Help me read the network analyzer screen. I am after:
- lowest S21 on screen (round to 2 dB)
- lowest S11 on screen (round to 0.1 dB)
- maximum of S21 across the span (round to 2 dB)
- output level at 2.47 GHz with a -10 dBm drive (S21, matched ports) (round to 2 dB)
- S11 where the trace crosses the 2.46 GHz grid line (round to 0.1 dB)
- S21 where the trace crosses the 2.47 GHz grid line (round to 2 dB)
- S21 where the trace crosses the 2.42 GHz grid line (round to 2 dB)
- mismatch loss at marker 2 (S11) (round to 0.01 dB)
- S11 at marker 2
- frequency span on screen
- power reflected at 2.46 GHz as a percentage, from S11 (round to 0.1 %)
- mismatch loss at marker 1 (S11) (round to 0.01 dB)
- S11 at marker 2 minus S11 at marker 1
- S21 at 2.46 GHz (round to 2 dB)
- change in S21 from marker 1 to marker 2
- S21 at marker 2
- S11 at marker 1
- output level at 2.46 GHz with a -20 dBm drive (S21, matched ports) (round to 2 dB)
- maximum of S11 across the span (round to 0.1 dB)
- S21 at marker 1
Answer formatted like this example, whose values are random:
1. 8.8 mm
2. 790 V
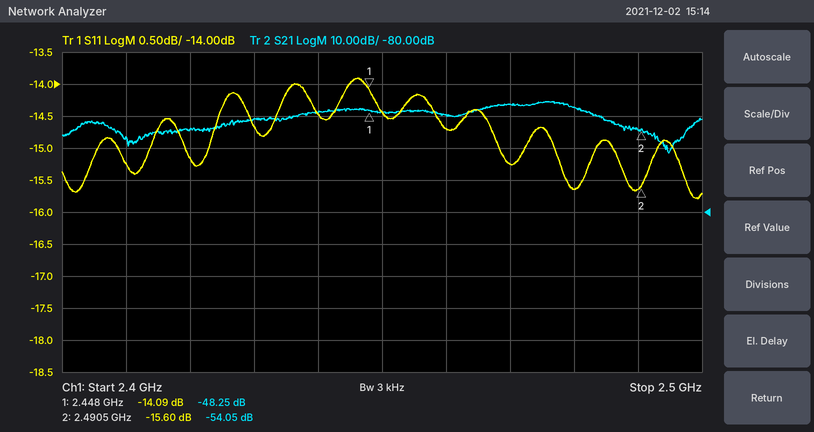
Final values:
1. -62 dB
2. -15.8 dB
3. -46 dB
4. -56 dBm
5. -14.7 dB
6. -46 dB
7. -54 dB
8. 0.12 dB
9. -15.60 dB
10. 100 MHz
11. 3.4 %
12. 0.17 dB
13. -1.51 dB
14. -50 dB
15. -5.80 dB
16. -54.05 dB
17. -14.09 dB
18. -70 dBm
19. -13.9 dB
20. -48.25 dB
